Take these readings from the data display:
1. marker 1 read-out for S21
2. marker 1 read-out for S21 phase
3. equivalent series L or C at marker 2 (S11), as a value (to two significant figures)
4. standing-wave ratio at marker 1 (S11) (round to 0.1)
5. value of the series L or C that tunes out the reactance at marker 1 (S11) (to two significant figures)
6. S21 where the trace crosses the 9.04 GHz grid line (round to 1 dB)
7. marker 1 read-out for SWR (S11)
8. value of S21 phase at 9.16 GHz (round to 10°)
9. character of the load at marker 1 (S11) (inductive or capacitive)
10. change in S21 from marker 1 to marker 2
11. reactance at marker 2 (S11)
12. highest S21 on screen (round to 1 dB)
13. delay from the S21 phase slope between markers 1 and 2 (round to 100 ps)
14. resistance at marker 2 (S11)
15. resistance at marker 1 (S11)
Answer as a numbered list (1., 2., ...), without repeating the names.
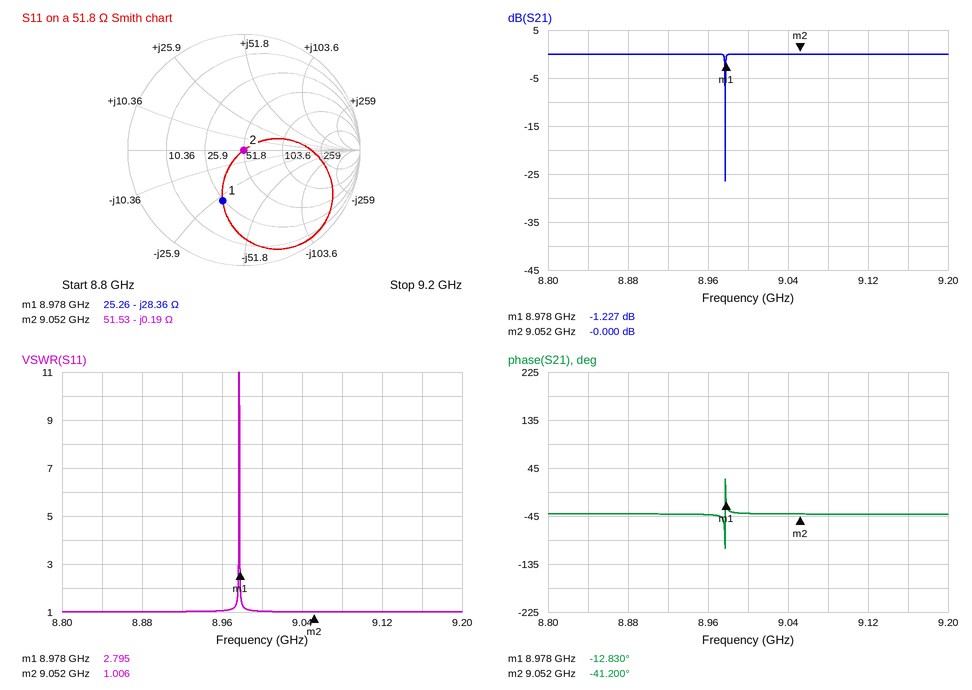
1. -1.227 dB
2. -12.830°
3. 93 pF
4. 2.8
5. 500 pH
6. 0 dB
7. 2.795
8. -40°
9. capacitive
10. 1.227 dB
11. -0.19 Ω
12. 0 dB
13. 1.1 ns
14. 51.53 Ω
15. 25.26 Ω
